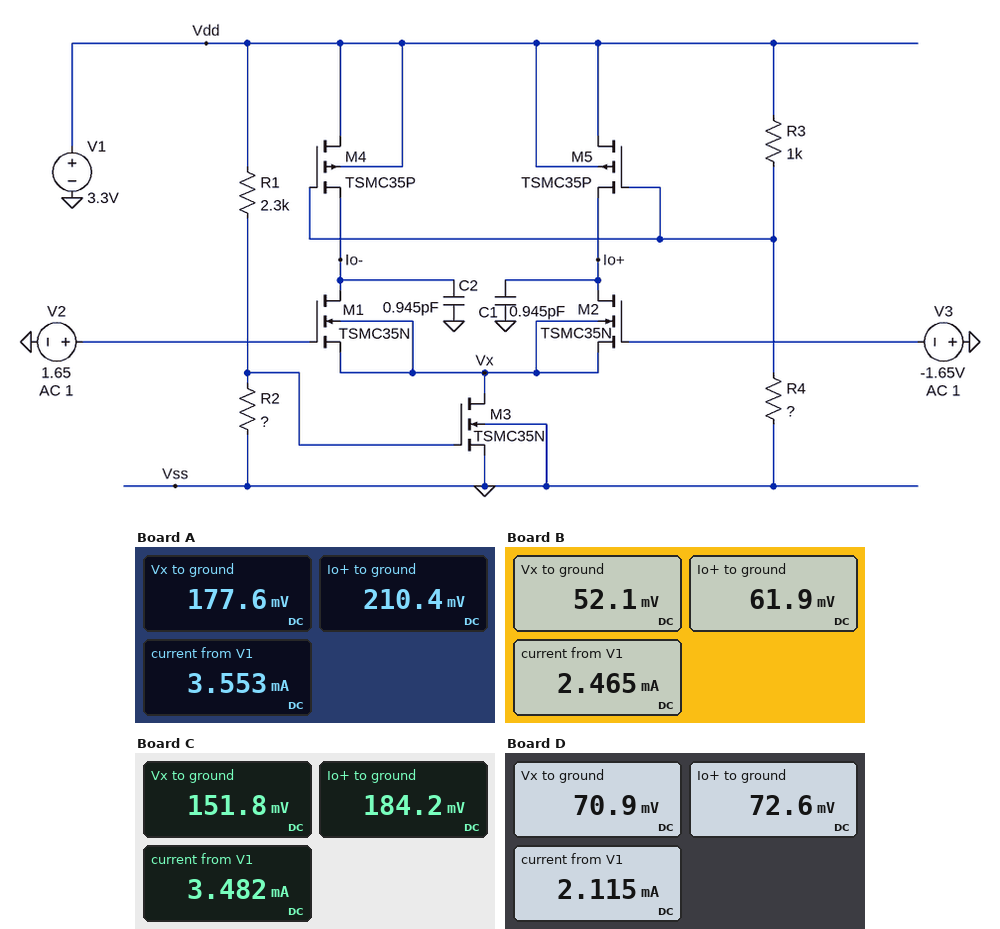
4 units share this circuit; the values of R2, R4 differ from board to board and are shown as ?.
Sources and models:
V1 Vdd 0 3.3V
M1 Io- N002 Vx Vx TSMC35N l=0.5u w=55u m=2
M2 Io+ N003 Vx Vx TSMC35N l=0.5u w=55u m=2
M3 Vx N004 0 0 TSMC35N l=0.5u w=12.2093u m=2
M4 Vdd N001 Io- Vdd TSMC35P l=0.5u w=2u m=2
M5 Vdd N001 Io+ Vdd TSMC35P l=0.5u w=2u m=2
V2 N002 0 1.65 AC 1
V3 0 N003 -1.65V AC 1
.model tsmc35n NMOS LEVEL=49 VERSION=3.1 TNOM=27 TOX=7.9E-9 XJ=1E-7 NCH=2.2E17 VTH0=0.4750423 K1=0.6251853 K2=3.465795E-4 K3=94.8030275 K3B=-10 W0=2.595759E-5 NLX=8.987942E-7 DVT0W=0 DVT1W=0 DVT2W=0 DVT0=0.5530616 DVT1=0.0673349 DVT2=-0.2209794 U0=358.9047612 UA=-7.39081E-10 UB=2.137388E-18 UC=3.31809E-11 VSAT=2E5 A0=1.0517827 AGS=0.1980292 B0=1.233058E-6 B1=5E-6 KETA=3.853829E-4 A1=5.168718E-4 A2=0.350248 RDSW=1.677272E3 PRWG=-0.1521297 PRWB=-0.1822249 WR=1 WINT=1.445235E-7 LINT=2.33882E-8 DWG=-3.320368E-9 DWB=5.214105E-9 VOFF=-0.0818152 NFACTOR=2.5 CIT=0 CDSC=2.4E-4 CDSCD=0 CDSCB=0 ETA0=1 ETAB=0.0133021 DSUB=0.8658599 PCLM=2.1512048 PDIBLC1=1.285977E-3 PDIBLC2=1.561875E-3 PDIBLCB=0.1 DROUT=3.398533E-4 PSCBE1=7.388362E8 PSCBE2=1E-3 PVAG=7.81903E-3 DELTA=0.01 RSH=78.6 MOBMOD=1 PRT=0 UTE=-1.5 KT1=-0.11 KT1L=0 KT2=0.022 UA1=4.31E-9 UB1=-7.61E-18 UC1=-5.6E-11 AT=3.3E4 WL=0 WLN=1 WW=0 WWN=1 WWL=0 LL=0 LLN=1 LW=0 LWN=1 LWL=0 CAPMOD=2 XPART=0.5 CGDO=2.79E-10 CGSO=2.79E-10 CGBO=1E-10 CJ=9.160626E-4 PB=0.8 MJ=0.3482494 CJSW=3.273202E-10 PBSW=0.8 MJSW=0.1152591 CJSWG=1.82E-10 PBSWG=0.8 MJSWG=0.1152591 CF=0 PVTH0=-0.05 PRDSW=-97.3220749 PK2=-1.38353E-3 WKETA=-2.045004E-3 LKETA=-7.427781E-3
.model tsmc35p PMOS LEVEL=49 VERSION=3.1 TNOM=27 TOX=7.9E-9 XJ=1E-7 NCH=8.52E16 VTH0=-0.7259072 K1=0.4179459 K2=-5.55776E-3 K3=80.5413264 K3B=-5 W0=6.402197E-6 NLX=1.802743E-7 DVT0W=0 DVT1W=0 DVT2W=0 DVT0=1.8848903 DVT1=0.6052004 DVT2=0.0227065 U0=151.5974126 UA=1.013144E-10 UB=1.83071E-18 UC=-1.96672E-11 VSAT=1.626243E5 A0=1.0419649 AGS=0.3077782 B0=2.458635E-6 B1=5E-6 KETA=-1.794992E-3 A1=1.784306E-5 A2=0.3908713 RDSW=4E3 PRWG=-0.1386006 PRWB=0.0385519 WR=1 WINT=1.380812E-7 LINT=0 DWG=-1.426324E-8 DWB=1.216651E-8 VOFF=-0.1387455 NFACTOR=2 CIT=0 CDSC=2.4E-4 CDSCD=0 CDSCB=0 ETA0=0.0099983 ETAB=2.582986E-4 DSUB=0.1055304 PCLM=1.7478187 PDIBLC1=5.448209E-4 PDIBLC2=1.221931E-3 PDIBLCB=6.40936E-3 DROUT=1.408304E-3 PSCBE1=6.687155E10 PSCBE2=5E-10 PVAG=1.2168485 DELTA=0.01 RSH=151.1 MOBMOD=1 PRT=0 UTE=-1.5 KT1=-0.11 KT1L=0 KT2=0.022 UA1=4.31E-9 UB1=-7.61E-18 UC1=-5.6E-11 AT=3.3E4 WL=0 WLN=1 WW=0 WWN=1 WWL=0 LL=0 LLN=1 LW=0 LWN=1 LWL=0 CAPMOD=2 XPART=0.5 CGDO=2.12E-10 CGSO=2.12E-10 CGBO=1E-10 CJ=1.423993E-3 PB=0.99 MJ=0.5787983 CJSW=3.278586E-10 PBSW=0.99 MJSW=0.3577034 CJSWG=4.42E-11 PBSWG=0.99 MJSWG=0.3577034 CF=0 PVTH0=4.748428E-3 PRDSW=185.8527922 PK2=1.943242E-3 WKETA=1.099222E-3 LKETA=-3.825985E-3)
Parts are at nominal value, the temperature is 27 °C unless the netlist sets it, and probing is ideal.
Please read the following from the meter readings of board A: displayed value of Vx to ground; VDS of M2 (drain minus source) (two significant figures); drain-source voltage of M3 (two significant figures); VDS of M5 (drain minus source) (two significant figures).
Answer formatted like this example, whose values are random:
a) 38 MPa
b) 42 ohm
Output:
a) 177.6 mV
b) 33 mV
c) 180 mV
d) 3.1 V
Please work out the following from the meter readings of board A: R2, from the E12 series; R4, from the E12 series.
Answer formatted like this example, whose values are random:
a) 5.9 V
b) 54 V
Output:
a) 1.8 kΩ
b) 470 Ω
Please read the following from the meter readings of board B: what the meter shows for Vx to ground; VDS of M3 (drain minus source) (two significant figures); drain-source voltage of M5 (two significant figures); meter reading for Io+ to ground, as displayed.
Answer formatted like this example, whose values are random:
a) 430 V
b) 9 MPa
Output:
a) 52.1 mV
b) 52 mV
c) 3.2 V
d) 61.9 mV
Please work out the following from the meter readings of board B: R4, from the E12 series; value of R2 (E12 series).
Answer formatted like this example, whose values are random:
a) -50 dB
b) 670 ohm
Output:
a) 1.2 kΩ
b) 1.8 kΩ
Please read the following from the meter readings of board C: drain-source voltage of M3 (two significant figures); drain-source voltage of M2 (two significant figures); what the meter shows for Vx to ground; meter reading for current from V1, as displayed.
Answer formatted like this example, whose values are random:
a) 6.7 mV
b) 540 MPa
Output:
a) 150 mV
b) 32 mV
c) 151.8 mV
d) 3.482 mA
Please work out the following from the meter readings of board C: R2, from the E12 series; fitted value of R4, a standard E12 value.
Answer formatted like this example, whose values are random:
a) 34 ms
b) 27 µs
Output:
a) 2.2 kΩ
b) 470 Ω
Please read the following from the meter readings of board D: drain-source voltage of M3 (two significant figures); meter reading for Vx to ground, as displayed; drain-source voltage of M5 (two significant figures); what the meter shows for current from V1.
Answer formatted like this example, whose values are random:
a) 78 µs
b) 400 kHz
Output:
a) 71 mV
b) 70.9 mV
c) 3.2 V
d) 2.115 mA
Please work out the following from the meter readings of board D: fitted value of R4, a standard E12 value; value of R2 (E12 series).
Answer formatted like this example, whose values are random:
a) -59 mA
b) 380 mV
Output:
a) 2.2 kΩ
b) 820 Ω
